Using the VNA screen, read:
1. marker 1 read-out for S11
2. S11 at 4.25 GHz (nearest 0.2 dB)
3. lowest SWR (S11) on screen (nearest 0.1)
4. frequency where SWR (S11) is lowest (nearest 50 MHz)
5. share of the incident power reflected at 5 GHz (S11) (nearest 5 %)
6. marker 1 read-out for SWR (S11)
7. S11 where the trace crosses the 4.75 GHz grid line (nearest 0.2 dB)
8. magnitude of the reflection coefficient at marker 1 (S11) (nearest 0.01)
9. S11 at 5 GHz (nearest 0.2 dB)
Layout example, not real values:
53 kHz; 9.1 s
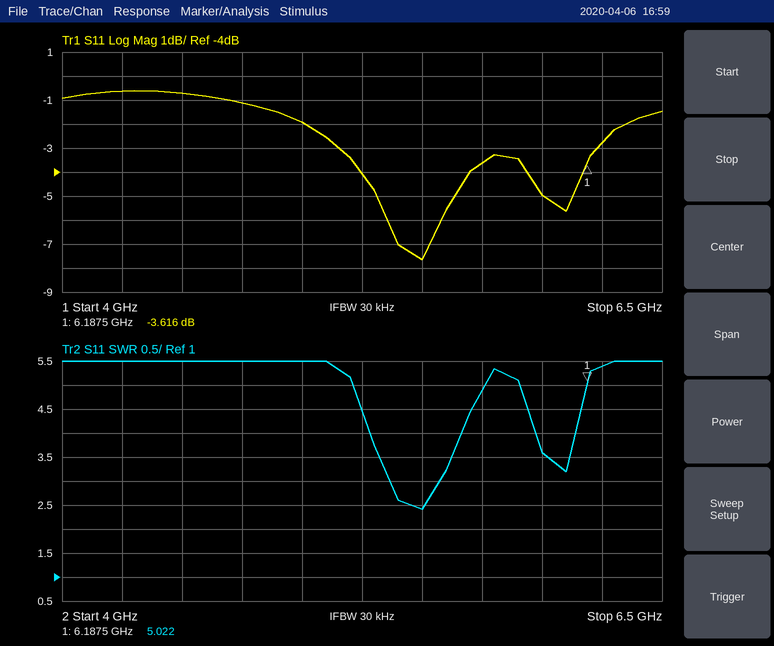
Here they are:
-3.616 dB; -0.6 dB; 2.4; 5.50 GHz; 65 %; 5.022; -1.2 dB; 0.66; -2.0 dB
